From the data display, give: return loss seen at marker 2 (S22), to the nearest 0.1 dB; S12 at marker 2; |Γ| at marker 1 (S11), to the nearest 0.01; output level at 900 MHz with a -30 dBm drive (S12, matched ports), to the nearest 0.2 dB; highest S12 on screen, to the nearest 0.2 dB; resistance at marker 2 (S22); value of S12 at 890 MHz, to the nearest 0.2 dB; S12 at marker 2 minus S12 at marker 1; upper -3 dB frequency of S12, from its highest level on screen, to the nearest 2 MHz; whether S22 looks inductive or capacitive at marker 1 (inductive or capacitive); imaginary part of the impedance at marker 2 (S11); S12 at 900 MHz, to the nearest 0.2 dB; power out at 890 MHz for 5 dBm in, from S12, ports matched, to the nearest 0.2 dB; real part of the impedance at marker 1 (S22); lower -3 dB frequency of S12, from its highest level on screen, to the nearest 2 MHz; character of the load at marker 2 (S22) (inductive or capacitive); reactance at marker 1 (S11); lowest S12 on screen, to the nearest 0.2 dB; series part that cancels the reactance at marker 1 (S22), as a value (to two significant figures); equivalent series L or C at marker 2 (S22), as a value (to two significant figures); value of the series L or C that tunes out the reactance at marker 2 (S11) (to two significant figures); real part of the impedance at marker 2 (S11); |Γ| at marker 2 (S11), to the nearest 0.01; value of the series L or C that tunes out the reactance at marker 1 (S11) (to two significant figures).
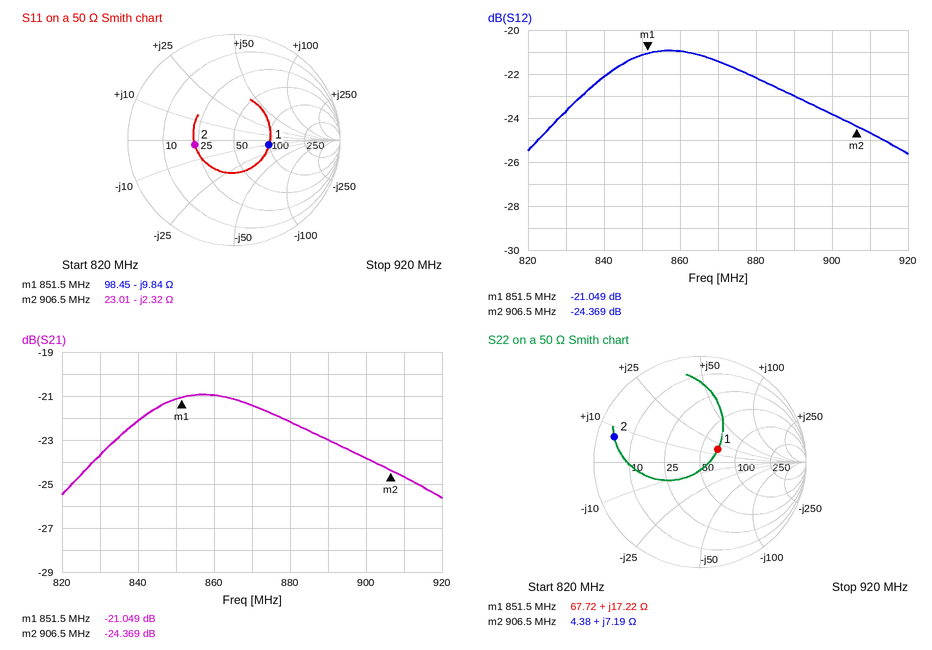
1.5 dB
-24.369 dB
0.33
-53.8 dBm
-21.0 dB
4.38 Ω
-23.0 dB
-3.320 dB
902 MHz
inductive
-2.32 Ω
-23.8 dB
-18.0 dBm
67.72 Ω
828 MHz
inductive
-9.84 Ω
-25.6 dB
11 pF
1.3 nH
410 pH
23.01 Ω
0.37
1.8 nH
